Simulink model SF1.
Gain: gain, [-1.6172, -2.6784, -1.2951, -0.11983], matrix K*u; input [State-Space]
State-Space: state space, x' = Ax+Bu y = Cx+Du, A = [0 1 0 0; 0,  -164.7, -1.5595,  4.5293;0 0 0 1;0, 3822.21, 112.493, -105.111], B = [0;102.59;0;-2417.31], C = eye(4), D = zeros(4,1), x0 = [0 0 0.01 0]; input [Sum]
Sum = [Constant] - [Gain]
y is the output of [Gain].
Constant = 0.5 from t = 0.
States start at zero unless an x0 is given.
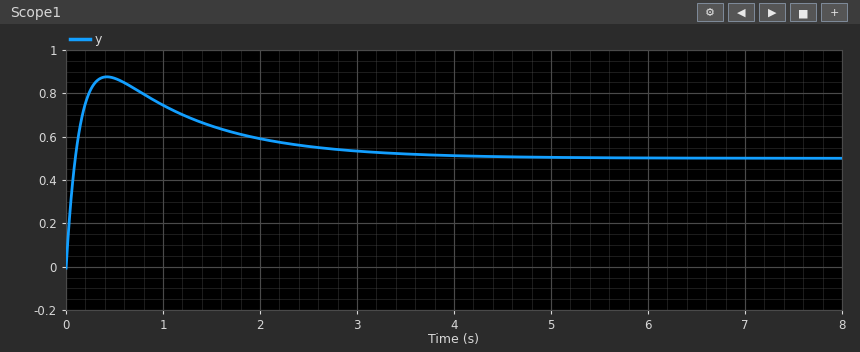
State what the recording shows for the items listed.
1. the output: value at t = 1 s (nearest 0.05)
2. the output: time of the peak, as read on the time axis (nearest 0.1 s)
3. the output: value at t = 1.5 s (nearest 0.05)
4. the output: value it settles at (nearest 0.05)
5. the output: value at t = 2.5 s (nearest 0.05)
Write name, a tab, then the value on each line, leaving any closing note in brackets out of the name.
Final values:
the output: value at t = 1 s	0.75
the output: time of the peak, as read on the time axis	0.4 s
the output: value at t = 1.5 s	0.65
the output: value it settles at	0.50
the output: value at t = 2.5 s	0.55
